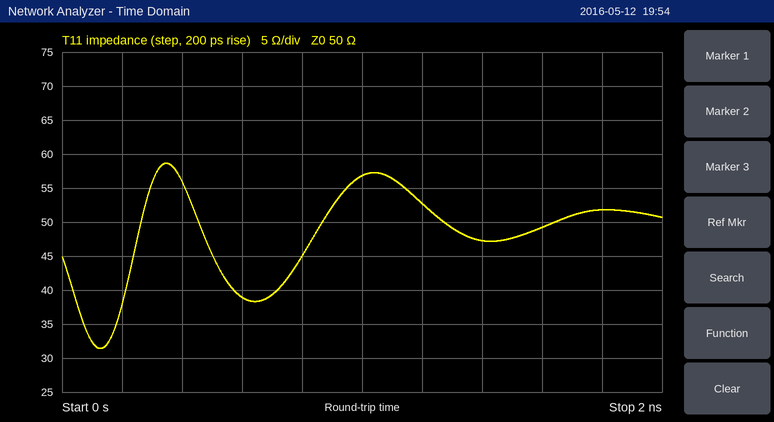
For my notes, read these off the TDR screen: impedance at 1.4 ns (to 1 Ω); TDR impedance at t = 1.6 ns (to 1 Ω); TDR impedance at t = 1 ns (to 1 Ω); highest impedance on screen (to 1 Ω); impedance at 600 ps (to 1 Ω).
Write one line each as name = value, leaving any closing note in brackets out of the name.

impedance at 1.4 ns = 47 Ω
TDR impedance at t = 1.6 ns = 49 Ω
TDR impedance at t = 1 ns = 57 Ω
highest impedance on screen = 59 Ω
impedance at 600 ps = 39 Ω
